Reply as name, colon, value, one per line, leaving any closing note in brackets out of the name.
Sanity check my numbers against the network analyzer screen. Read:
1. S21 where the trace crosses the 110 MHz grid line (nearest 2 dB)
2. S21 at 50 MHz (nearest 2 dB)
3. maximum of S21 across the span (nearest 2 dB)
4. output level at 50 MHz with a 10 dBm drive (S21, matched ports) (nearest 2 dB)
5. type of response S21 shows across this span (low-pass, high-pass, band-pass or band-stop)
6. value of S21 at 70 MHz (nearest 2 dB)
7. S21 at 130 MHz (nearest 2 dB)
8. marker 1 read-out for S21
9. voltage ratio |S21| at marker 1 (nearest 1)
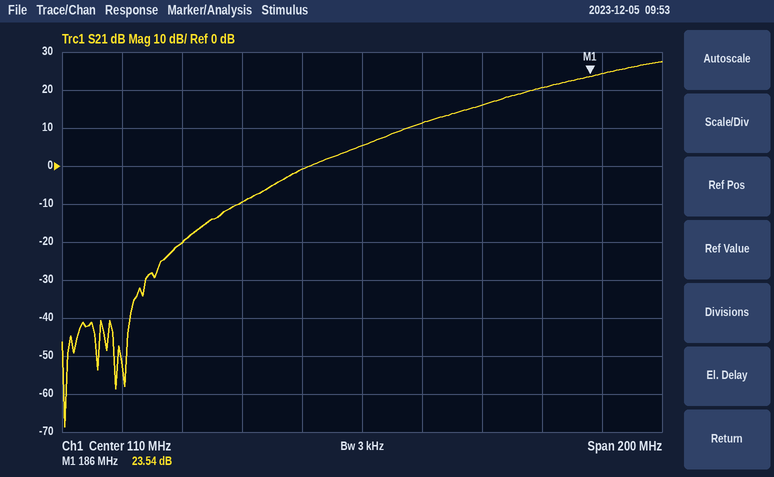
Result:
S21 where the trace crosses the 110 MHz grid line: 6 dB
S21 at 50 MHz: -20 dB
maximum of S21 across the span: 28 dB
output level at 50 MHz with a 10 dBm drive (S21, matched ports): -10 dBm
type of response S21 shows across this span: high-pass
value of S21 at 70 MHz: -10 dB
S21 at 130 MHz: 12 dB
marker 1 read-out for S21: 23.54 dB
voltage ratio |S21| at marker 1: 15
